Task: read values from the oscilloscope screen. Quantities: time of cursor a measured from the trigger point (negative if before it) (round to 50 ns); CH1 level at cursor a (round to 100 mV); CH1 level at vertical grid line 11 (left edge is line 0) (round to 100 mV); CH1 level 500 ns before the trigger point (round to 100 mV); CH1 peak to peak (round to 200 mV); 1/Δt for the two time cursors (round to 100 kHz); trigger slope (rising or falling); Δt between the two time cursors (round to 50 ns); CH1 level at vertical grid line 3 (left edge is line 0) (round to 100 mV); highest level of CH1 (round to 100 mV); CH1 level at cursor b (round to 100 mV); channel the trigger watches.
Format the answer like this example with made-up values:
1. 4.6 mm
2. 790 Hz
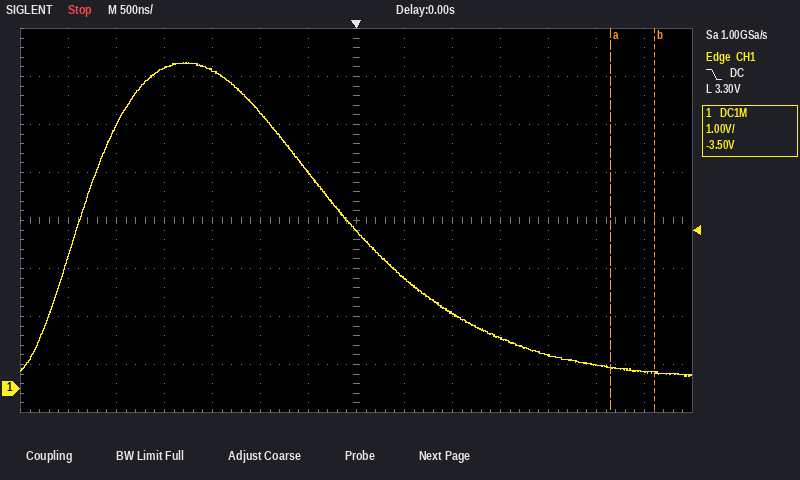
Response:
1. +2.65 µs
2. 400 mV
3. 700 mV
4. 4.5 V
5. 6.6 V
6. 2.2 MHz
7. falling
8. 450 ns
9. 6.7 V
10. 6.8 V
11. 300 mV
12. CH1
